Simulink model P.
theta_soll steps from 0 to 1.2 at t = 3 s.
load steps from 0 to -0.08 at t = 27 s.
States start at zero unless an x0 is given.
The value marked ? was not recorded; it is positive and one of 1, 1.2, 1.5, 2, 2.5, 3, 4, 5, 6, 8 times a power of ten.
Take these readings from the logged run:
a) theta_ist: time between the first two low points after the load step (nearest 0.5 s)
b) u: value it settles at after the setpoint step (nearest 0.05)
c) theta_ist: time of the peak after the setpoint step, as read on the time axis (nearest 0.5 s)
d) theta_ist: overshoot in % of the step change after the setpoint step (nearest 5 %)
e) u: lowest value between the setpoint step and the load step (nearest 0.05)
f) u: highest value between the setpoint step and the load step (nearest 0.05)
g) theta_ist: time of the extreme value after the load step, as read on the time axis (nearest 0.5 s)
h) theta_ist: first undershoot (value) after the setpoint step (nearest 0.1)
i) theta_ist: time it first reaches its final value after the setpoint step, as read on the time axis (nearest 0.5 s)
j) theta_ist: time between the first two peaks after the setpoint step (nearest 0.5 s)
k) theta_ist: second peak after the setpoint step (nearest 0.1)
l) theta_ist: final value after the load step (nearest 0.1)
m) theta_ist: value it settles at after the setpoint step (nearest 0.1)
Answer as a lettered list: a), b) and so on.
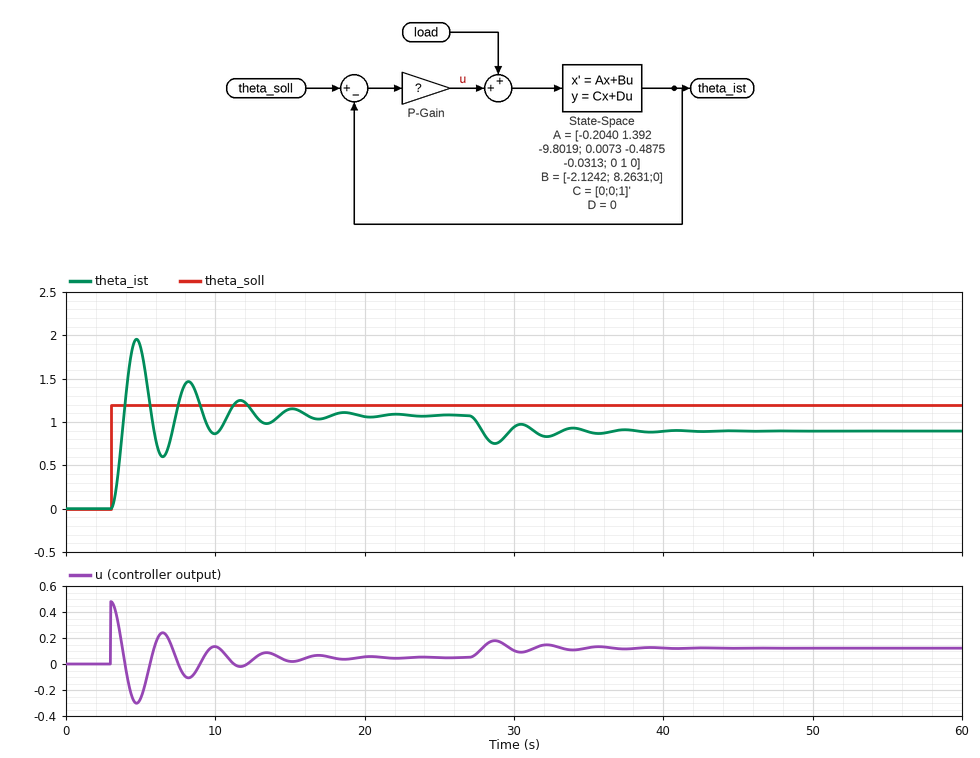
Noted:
a) 3.5 s
b) 0.05
c) 4.5 s
d) 80 %
e) -0.30
f) 0.50
g) 28.5 s
h) 0.6
i) 4.0 s
j) 3.5 s
k) 1.5
l) 0.9
m) 1.1
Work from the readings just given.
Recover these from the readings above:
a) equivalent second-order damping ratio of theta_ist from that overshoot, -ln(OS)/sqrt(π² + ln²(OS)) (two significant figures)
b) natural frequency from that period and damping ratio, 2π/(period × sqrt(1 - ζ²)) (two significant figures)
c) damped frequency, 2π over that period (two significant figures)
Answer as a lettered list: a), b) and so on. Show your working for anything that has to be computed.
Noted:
a) ln(0.8) = -0.223; 0.223 / sqrt(9.870 + 0.050) = 0.071
b) 2π / (3.5 × sqrt(1 - 0.071²)) = 1.8 rad/s
c) 2π / 3.5 = 1.8 rad/s
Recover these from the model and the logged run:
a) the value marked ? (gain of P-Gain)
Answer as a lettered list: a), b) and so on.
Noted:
a) 0.4
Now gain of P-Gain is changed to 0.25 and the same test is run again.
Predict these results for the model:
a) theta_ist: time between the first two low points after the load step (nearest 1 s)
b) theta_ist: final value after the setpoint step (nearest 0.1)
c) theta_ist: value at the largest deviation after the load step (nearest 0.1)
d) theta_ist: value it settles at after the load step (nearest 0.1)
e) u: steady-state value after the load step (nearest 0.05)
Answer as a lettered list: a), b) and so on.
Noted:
a) 4 s
b) 1.0
c) 0.5
d) 0.7
e) 0.10
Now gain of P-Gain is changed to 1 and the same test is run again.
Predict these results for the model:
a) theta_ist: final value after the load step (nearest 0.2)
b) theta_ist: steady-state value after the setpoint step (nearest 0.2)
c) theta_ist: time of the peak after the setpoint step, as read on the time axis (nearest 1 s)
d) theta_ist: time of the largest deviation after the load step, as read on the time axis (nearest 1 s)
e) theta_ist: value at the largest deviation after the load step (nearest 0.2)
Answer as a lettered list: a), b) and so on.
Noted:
a) 1.0
b) 1.2
c) 4 s
d) 28 s
e) 1.0
